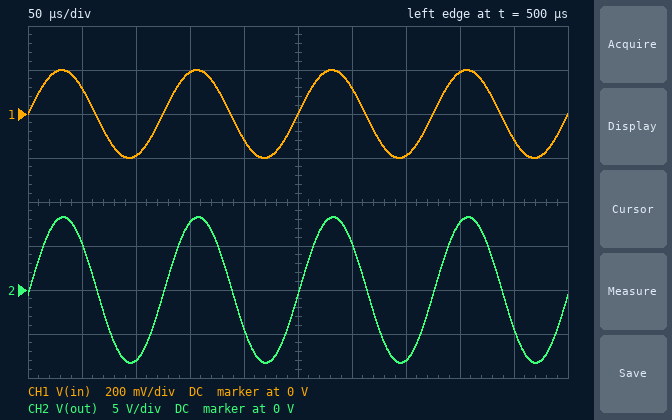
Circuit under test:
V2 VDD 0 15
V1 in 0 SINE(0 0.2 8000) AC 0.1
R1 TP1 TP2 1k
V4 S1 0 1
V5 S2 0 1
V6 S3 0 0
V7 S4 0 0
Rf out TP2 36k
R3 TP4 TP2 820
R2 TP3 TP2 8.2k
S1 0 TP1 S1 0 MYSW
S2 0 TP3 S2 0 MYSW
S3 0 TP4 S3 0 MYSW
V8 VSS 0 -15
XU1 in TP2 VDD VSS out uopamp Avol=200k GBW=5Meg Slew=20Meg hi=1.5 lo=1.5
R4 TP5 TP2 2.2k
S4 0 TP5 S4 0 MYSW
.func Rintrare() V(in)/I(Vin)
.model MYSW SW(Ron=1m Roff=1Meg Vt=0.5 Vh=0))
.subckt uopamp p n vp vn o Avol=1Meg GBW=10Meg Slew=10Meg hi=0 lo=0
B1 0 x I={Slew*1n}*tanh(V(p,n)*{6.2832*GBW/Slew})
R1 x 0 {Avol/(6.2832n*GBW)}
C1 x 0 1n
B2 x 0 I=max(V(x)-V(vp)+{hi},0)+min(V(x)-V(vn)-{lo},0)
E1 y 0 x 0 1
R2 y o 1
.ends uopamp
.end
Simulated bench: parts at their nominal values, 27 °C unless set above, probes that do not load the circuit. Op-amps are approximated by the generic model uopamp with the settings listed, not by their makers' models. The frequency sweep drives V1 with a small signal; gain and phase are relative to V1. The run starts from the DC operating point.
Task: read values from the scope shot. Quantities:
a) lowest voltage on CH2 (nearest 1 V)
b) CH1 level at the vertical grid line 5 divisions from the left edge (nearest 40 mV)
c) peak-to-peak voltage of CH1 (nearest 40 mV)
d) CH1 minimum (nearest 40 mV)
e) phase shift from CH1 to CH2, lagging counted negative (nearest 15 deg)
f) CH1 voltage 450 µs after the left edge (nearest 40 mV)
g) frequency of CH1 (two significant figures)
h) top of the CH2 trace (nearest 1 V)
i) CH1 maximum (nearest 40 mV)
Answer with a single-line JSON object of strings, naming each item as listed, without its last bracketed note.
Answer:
{"lowest voltage on CH2": "-8 V", "CH1 level at the vertical grid line 5 divisions from the left edge": "0 V", "peak-to-peak voltage of CH1": "400 mV", "CH1 minimum": "-200 mV", "phase shift from CH1 to CH2, lagging counted negative": "0 deg", "CH1 voltage 450 µs after the left edge": "-120 mV", "frequency of CH1": "8.0 kHz", "top of the CH2 trace": "8 V", "CH1 maximum": "200 mV"}
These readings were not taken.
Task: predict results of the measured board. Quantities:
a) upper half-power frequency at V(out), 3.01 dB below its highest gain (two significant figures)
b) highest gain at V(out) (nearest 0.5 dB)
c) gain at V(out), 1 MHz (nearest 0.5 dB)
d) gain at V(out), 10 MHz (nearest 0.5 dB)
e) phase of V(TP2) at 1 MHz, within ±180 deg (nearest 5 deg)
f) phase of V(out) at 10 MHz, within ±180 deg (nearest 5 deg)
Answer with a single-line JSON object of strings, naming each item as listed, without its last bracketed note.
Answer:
{"upper half-power frequency at V(out), 3.01 dB below its highest gain": "4.4 MHz", "highest gain at V(out)": "1.0 dB", "gain at V(out), 1 MHz": "1.0 dB", "gain at V(out), 10 MHz": "-7.0 dB", "phase of V(TP2) at 1 MHz, within ±180 deg": "-15 deg", "phase of V(out) at 10 MHz, within ±180 deg": "-65 deg"}
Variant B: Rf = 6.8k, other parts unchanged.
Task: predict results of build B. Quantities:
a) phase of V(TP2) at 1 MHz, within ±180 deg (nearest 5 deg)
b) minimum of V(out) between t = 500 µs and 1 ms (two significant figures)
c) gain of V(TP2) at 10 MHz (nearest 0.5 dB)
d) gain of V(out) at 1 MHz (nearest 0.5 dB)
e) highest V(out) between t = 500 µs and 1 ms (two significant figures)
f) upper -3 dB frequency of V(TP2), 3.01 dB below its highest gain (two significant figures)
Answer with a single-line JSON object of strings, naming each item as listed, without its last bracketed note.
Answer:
{"phase of V(TP2) at 1 MHz, within ±180 deg": "-10 deg", "minimum of V(out) between t = 500 µs and 1 ms": "-1.7 V", "gain of V(TP2) at 10 MHz": "-7.0 dB", "gain of V(out) at 1 MHz": "0 dB", "highest V(out) between t = 500 µs and 1 ms": "1.7 V", "upper -3 dB frequency of V(TP2), 3.01 dB below its highest gain": "4.9 MHz"}
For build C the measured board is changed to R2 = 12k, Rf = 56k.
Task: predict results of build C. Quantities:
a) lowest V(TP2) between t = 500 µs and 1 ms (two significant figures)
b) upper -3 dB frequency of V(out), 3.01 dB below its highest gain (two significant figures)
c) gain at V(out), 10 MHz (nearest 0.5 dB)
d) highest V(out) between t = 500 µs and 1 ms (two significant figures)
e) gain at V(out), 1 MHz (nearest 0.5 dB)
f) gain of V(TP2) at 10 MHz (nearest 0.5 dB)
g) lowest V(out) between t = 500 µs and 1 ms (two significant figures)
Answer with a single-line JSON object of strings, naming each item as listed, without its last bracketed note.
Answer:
{"lowest V(TP2) between t = 500 µs and 1 ms": "-200 mV", "upper -3 dB frequency of V(out), 3.01 dB below its highest gain": "4.1 MHz", "gain at V(out), 10 MHz": "-6.5 dB", "highest V(out) between t = 500 µs and 1 ms": "12 V", "gain at V(out), 1 MHz": "1.5 dB", "gain of V(TP2) at 10 MHz": "-8.5 dB", "lowest V(out) between t = 500 µs and 1 ms": "-12 V"}
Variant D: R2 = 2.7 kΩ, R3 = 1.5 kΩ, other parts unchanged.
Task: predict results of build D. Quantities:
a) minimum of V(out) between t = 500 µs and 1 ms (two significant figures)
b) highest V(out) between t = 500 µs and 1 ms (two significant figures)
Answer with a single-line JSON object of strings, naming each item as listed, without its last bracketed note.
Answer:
{"minimum of V(out) between t = 500 µs and 1 ms": "-10 V", "highest V(out) between t = 500 µs and 1 ms": "10 V"}
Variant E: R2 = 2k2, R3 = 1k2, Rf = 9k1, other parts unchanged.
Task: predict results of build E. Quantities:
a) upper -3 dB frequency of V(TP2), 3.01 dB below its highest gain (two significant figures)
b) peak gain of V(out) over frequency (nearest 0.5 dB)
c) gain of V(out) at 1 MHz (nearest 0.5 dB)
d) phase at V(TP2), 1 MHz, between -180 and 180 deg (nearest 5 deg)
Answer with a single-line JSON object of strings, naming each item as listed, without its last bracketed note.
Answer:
{"upper -3 dB frequency of V(TP2), 3.01 dB below its highest gain": "4.8 MHz", "peak gain of V(out) over frequency": "0.5 dB", "gain of V(out) at 1 MHz": "0 dB", "phase at V(TP2), 1 MHz, between -180 and 180 deg": "-10 deg"}
